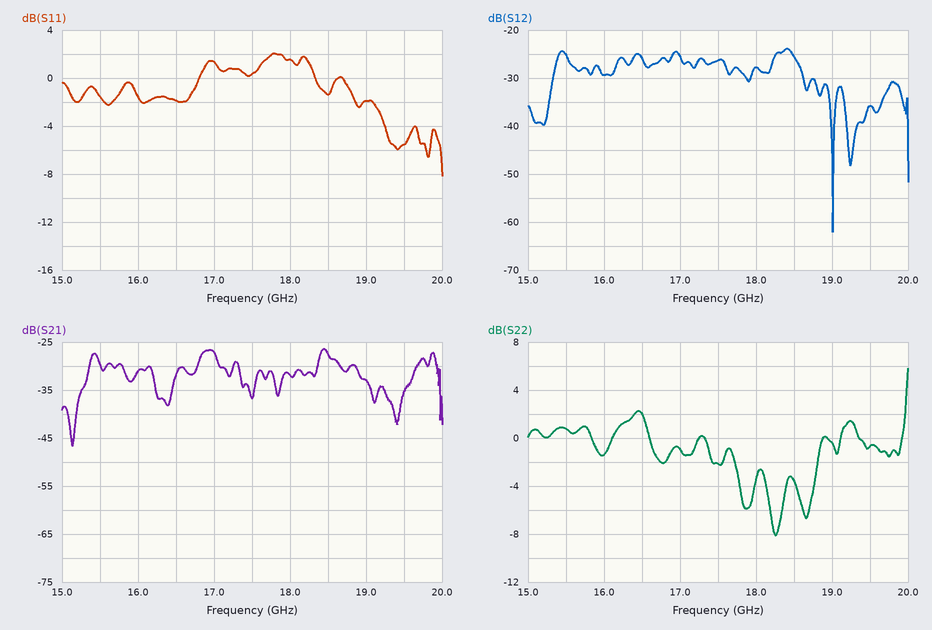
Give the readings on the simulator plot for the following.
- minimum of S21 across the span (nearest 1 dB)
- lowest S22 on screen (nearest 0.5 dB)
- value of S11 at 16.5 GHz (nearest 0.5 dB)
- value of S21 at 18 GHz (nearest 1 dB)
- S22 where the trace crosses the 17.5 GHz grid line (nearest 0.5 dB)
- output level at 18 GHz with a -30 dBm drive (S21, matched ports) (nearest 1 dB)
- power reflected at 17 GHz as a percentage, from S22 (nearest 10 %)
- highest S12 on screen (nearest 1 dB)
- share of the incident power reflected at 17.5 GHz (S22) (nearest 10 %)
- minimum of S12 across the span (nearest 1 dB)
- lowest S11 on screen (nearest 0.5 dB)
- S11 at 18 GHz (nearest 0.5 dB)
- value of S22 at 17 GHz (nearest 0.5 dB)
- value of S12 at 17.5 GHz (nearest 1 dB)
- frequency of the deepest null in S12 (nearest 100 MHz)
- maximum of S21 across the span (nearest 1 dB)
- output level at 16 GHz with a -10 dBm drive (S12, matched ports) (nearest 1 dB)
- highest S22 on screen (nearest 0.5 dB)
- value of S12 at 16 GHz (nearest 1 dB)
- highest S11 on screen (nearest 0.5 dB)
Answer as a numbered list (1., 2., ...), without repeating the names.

1. -47 dB
2. -8.0 dB
3. -2.0 dB
4. -32 dB
5. -2.0 dB
6. -62 dBm
7. 80 %
8. -24 dB
9. 60 %
10. -62 dB
11. -8.0 dB
12. 1.5 dB
13. -1.0 dB
14. -26 dB
15. 19.0 GHz
16. -26 dB
17. -39 dBm
18. 6.0 dB
19. -29 dB
20. 2.0 dB
